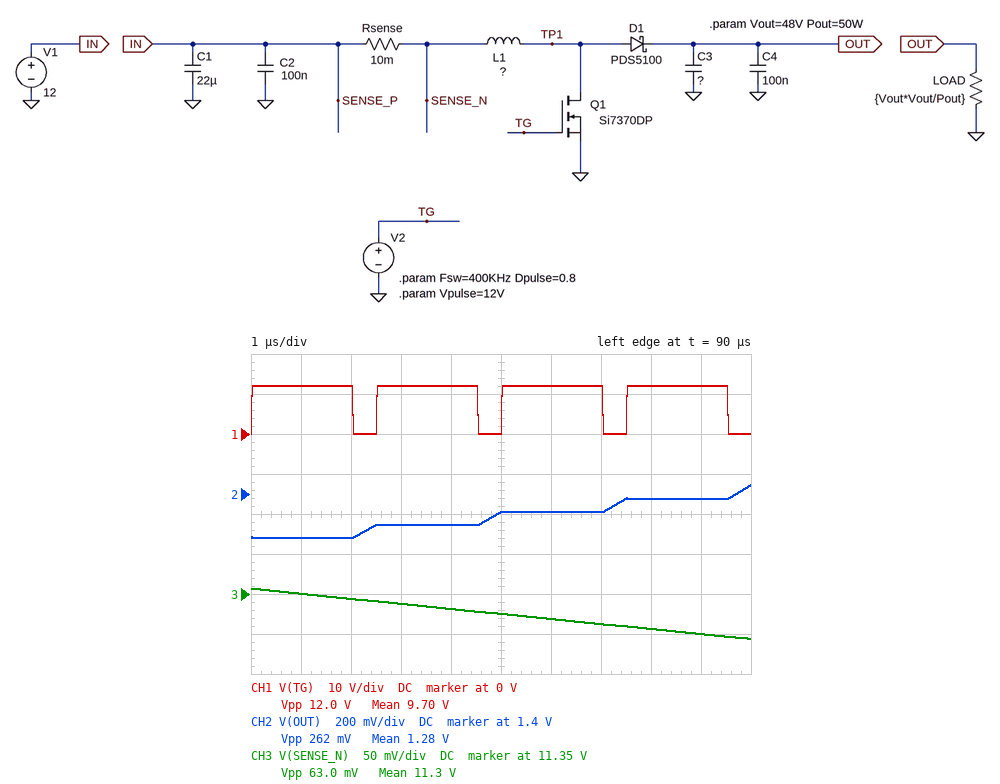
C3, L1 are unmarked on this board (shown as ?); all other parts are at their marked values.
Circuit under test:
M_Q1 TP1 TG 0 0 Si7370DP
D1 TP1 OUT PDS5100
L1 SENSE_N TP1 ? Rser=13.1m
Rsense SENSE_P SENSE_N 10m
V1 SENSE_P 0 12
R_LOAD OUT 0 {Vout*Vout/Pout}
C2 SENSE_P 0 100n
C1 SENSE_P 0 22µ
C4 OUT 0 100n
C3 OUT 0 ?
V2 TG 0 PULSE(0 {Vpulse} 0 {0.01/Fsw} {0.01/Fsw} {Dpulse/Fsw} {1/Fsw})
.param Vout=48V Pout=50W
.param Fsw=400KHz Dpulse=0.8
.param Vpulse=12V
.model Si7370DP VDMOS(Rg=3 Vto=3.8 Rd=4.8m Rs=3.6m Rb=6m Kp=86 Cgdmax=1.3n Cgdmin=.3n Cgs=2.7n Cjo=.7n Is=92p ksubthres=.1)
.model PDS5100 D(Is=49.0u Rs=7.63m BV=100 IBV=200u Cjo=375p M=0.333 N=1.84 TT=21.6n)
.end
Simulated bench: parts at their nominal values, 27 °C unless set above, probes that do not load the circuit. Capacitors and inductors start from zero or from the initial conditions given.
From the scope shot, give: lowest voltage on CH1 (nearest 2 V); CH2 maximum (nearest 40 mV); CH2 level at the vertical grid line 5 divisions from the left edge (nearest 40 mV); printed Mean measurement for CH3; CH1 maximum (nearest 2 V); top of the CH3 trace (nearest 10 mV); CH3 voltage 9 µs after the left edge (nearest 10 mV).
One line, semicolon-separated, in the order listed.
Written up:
0 V; 1.44 V; 1.32 V; 11.3 V; 12 V; 11.36 V; 11.30 V
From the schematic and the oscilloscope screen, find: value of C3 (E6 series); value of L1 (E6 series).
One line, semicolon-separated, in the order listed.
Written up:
470 µF; 15 µH
